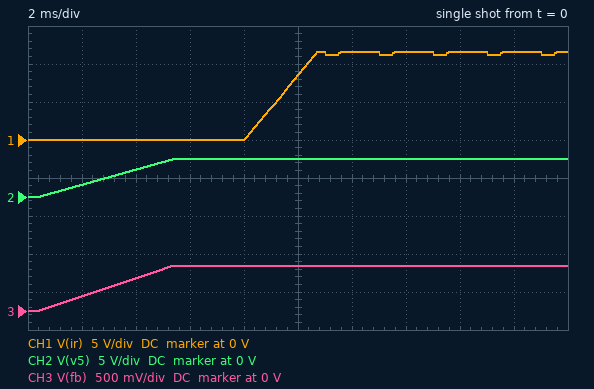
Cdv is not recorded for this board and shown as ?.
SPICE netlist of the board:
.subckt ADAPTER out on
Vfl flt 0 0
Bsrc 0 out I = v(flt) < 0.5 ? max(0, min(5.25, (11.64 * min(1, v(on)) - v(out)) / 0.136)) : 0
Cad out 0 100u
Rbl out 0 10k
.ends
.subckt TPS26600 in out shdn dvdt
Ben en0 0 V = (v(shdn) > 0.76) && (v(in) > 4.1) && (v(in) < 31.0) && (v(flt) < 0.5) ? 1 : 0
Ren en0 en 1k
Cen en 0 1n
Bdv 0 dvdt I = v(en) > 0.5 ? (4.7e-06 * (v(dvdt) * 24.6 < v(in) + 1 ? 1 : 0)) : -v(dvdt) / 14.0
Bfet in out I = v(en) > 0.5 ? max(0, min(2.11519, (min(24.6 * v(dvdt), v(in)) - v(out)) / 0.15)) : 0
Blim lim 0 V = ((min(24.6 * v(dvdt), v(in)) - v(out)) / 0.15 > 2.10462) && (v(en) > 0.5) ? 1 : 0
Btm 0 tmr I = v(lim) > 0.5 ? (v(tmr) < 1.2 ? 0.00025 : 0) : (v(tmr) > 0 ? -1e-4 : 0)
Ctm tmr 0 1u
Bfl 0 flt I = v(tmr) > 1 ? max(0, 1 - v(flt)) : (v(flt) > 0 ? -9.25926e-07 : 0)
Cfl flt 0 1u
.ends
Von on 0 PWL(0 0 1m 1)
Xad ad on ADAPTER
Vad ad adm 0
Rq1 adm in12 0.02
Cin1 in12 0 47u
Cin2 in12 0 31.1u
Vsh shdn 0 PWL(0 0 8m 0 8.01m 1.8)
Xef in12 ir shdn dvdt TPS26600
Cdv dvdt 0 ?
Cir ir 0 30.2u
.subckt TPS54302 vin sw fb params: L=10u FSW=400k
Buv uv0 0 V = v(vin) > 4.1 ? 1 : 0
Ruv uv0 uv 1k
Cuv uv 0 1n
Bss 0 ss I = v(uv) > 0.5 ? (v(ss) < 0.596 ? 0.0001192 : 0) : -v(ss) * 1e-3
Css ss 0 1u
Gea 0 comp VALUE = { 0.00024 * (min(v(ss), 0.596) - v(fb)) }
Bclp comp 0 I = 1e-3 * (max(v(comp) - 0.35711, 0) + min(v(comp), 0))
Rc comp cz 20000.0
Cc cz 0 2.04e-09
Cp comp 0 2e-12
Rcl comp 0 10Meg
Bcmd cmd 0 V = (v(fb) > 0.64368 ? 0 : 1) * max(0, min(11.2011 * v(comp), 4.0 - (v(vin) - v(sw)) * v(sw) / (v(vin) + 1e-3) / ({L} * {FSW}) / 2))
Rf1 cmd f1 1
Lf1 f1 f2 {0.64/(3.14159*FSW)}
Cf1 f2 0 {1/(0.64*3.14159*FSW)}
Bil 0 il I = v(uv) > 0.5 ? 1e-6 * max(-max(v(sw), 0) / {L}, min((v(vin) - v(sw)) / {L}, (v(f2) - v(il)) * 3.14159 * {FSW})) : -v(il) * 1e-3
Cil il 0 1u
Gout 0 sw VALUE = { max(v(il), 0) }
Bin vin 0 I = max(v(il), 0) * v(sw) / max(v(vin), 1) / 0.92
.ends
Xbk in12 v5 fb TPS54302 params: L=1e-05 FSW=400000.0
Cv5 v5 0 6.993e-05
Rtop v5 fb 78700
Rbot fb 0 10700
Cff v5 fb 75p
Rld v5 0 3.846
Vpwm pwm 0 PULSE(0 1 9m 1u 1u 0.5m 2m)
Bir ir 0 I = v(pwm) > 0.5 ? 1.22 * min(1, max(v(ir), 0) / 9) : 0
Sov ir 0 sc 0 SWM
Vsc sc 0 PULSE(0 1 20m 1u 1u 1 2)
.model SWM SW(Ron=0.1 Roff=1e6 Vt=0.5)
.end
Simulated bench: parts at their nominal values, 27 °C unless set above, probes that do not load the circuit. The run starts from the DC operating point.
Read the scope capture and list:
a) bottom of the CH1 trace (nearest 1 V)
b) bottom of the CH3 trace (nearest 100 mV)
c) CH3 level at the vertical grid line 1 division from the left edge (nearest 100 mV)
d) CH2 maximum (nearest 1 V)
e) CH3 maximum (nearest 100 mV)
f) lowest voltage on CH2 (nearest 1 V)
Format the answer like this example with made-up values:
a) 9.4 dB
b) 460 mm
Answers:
a) 0 V
b) 0 V
c) 200 mV
d) 5 V
e) 600 mV
f) 0 V
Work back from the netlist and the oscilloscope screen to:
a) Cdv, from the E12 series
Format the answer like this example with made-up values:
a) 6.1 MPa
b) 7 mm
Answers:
a) 27 nF
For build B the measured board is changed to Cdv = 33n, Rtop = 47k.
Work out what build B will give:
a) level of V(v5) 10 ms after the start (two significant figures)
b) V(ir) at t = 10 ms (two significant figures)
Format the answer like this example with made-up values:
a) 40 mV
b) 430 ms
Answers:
a) 3.2 V
b) 7.0 V
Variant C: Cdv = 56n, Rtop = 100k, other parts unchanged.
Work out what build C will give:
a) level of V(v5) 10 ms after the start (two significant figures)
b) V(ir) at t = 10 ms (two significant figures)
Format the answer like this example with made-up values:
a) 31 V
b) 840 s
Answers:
a) 6.2 V
b) 4.1 V
